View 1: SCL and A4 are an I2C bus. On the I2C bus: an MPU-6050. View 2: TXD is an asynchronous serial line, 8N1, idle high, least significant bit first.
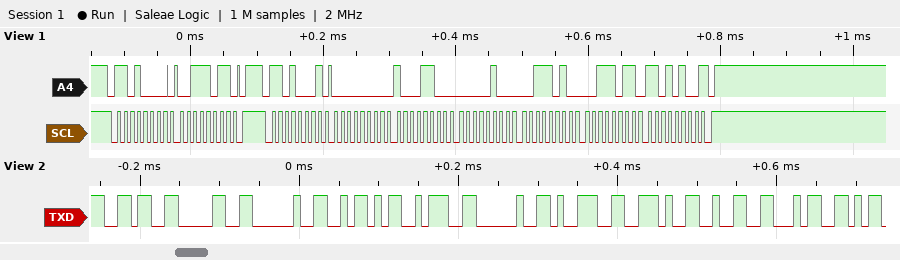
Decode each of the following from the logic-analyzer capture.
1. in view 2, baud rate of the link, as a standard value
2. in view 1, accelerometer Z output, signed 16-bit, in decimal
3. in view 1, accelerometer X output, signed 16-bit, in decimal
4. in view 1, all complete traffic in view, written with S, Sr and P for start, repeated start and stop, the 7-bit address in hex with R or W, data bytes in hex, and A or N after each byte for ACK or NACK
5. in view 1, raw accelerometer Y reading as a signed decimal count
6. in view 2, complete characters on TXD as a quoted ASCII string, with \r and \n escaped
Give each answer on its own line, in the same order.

115200 baud
15316
140
S 68W A 3B A P S 68R A 00 A 8C A 04 A 3A A 3B A D4 N P
1082
"60 Z: 9.24"
